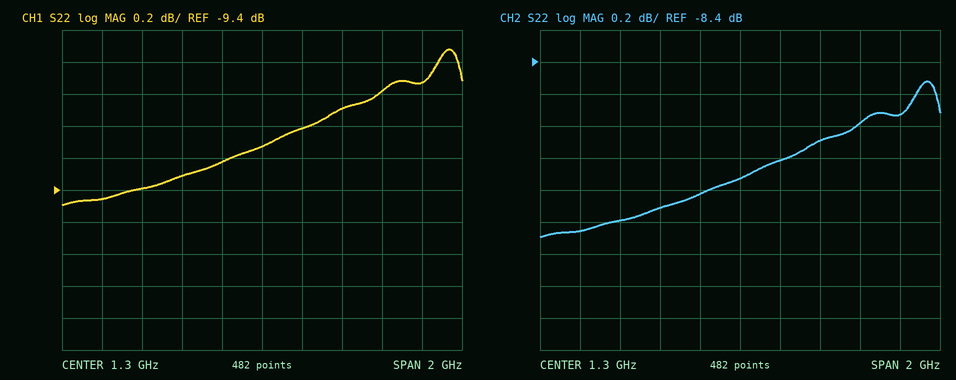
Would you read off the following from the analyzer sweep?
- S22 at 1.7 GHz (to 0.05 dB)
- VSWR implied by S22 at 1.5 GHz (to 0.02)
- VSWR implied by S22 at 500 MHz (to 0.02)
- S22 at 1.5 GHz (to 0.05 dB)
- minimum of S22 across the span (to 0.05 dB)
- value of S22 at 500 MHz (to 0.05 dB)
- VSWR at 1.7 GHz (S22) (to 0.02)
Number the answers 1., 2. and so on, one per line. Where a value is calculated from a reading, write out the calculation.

1. -8.90 dB
2. |Γ| = 10^(-9/20) = 0.3548; VSWR = (1 + 0.3548)/(1 − 0.3548) ≈ 2.10
3. |Γ| = 10^(-9.45/20) = 0.3369; VSWR = (1 + 0.3369)/(1 − 0.3369) ≈ 2.02
4. -9.00 dB
5. -9.50 dB
6. -9.45 dB
7. |Γ| = 10^(-8.9/20) = 0.3589; VSWR = (1 + 0.3589)/(1 − 0.3589) ≈ 2.12
